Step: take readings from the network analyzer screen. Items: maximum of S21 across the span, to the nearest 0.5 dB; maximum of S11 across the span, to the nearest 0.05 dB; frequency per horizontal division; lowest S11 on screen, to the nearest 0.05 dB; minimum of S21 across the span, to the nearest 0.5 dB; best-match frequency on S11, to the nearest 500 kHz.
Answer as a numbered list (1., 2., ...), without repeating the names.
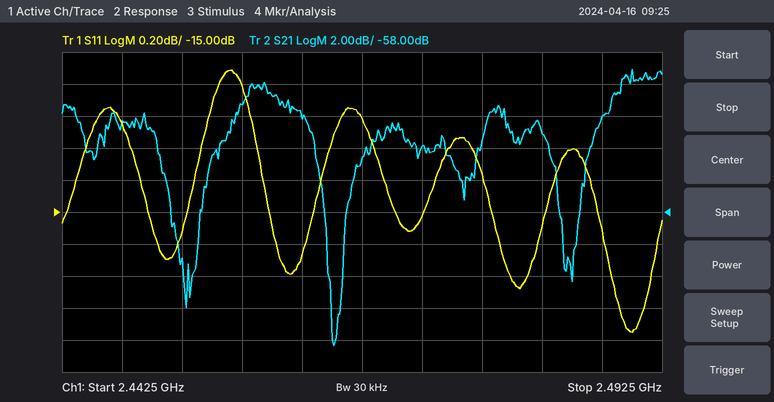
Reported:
1. -49.0 dB
2. -14.10 dB
3. 5 MHz
4. -15.75 dB
5. -66.5 dB
6. 2.4900 GHz
